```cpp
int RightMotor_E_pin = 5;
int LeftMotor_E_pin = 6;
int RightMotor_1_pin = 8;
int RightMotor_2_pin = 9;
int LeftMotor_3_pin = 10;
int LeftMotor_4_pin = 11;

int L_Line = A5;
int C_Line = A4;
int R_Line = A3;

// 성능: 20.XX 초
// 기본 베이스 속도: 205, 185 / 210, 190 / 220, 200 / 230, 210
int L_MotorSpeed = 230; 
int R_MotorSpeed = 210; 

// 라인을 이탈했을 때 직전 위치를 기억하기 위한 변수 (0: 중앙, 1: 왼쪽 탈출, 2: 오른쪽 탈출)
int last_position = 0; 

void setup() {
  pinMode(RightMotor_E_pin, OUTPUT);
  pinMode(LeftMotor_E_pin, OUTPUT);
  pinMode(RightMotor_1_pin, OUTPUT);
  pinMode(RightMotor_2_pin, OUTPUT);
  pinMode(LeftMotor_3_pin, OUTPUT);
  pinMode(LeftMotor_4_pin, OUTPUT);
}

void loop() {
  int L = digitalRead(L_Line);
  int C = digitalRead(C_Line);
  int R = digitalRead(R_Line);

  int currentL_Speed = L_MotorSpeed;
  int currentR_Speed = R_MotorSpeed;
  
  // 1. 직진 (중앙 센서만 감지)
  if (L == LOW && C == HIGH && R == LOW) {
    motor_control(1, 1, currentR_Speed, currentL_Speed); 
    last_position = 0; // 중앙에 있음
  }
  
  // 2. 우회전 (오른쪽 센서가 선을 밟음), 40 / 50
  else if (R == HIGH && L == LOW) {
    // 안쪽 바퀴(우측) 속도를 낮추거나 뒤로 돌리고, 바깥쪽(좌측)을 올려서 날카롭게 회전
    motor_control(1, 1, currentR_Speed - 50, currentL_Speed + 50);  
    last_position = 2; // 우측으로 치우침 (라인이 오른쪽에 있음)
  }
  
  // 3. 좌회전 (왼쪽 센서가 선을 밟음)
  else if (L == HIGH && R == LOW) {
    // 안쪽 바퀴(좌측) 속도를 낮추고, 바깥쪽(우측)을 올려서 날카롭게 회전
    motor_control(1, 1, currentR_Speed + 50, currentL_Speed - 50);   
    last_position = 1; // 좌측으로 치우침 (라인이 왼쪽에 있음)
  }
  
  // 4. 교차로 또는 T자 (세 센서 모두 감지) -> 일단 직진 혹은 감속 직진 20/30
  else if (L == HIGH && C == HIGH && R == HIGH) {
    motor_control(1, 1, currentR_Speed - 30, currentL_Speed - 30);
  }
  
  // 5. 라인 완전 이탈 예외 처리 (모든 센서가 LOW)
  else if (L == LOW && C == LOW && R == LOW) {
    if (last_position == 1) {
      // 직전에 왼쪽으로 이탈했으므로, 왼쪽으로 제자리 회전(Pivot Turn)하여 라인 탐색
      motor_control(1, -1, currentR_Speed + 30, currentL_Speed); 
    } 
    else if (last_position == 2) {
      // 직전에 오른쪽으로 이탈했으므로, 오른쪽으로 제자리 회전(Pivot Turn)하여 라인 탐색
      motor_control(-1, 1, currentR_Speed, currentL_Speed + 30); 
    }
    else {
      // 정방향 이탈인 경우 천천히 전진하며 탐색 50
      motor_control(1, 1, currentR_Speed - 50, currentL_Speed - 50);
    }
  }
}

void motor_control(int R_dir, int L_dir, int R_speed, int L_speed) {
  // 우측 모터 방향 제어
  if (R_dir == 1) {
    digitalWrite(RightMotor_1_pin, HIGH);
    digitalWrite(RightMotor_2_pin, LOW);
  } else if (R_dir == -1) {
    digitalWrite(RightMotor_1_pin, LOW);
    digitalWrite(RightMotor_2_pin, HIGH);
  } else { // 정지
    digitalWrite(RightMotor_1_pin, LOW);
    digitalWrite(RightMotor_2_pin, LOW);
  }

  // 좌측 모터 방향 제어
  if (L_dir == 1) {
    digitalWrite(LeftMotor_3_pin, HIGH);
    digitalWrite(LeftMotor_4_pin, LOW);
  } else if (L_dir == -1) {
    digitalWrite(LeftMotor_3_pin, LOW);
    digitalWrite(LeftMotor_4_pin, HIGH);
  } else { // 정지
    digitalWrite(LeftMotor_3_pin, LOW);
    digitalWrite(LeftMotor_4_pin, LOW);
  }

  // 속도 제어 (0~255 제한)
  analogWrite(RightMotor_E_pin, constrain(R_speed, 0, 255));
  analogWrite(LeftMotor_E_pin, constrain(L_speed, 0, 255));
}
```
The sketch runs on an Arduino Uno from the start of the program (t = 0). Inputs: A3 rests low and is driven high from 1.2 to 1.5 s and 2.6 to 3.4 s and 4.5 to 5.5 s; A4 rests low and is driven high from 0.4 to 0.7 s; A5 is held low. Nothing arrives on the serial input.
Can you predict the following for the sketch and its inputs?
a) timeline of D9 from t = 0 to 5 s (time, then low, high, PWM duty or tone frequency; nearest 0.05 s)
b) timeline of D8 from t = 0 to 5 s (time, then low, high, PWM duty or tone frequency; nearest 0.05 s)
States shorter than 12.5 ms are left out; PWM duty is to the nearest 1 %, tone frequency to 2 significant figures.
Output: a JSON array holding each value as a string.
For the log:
["0 s low; 1.5 s high; 2.6 s low; 3.4 s high; 4.5 s low", "0 s high; 1.5 s low; 2.6 s high; 3.4 s low; 4.5 s high"]
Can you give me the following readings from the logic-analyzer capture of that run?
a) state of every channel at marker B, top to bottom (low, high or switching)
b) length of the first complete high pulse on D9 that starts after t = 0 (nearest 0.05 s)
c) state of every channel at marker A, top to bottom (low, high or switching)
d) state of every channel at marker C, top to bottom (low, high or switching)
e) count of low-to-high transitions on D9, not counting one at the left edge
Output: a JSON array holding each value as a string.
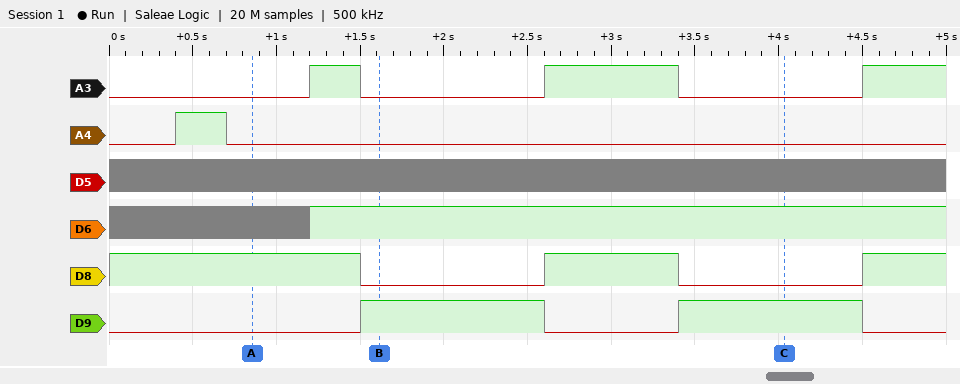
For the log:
["A3 low, A4 low, D5 switching, D6 high, D8 low, D9 high", "1.10 s", "A3 low, A4 low, D5 switching, D6 switching, D8 high, D9 low", "A3 low, A4 low, D5 switching, D6 high, D8 low, D9 high", "2"]
